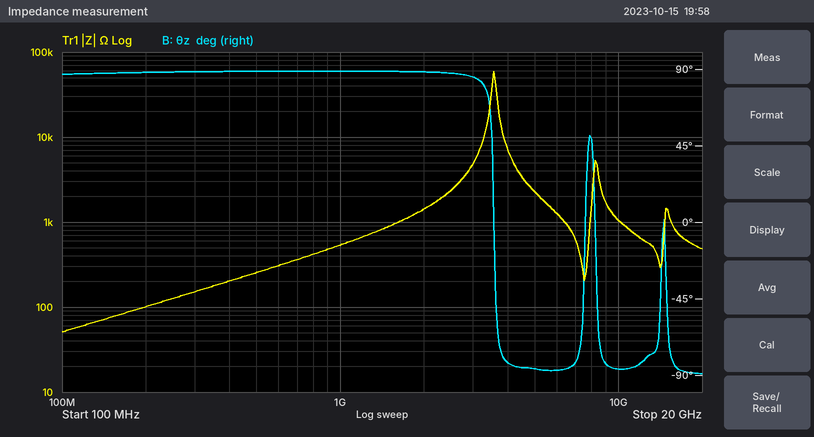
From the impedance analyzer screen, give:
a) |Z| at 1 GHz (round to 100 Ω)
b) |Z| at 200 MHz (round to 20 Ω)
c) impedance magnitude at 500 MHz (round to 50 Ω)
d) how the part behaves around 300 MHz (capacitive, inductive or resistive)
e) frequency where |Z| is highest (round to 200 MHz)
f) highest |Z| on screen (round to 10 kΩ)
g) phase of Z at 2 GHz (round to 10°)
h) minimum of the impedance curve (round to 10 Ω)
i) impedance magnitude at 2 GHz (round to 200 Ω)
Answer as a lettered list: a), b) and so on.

a) 500 Ω
b) 100 Ω
c) 250 Ω
d) inductive
e) 3.6 GHz
f) 60 kΩ
g) 90°
h) 50 Ω
i) 1.4 kΩ
